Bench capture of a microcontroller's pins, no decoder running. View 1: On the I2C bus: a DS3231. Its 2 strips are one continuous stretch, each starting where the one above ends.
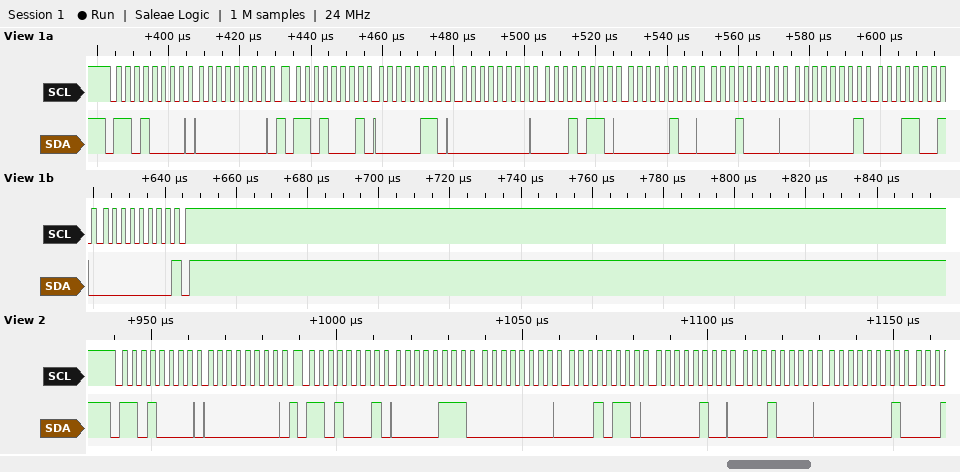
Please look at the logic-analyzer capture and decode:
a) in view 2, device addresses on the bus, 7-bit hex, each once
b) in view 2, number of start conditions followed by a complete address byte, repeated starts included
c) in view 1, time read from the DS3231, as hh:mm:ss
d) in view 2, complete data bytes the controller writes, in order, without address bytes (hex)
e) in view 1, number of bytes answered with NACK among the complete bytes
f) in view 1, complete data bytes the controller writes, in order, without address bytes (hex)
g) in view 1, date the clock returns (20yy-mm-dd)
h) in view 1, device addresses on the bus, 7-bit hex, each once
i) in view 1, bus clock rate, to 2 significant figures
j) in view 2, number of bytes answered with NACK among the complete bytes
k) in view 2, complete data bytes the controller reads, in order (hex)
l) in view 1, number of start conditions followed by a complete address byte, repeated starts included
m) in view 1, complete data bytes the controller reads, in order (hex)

0x68
2
16:00:06
00
1
00
2019-01-10
0x68
400 kHz
0
07 00 16 04 10 01
2
06 00 16 04 10 01 19 00
